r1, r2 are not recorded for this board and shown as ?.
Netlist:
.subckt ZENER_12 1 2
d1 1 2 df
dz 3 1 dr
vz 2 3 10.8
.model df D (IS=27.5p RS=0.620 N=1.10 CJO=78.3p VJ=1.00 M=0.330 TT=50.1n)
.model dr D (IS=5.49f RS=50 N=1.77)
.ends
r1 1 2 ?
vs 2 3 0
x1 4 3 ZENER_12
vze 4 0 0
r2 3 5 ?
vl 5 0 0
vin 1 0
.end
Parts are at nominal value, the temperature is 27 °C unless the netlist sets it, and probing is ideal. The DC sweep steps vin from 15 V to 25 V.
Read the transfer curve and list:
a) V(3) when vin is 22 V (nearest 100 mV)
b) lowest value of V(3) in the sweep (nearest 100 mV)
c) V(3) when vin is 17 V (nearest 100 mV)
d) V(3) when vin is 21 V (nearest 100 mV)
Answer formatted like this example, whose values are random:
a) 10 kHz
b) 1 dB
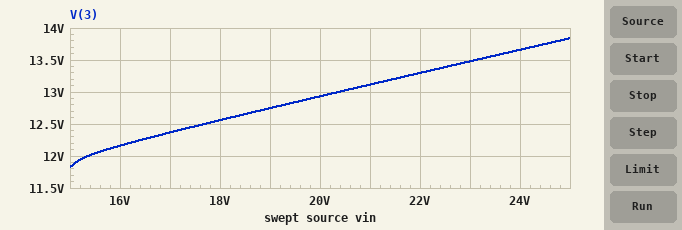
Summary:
a) 13.3 V
b) 11.8 V
c) 12.4 V
d) 13.1 V
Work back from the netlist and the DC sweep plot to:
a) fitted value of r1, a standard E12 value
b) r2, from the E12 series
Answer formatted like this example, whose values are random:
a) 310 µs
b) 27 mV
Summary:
a) 220 Ω
b) 820 Ω
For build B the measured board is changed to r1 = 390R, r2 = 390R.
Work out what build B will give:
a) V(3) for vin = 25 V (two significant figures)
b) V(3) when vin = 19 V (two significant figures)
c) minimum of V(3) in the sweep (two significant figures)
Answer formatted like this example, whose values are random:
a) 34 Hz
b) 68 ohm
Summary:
a) 12 V
b) 9.5 V
c) 7.5 V
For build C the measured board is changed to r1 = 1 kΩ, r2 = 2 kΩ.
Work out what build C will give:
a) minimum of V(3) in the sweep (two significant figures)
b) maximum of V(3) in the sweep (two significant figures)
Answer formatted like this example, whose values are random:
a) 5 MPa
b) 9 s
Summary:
a) 10 V
b) 12 V
